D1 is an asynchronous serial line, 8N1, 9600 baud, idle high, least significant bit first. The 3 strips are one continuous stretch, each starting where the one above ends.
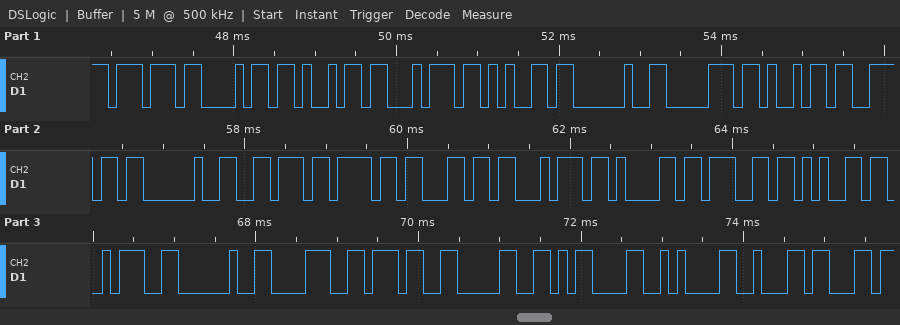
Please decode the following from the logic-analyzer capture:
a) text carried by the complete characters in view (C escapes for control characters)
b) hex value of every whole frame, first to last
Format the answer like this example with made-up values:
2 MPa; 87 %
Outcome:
"white pin voltage: 870\r\nb"; 77 68 69 74 65 20 70 69 6E 20 76 6F 6C 74 61 67 65 3A 20 38 37 30 0D 0A 62
